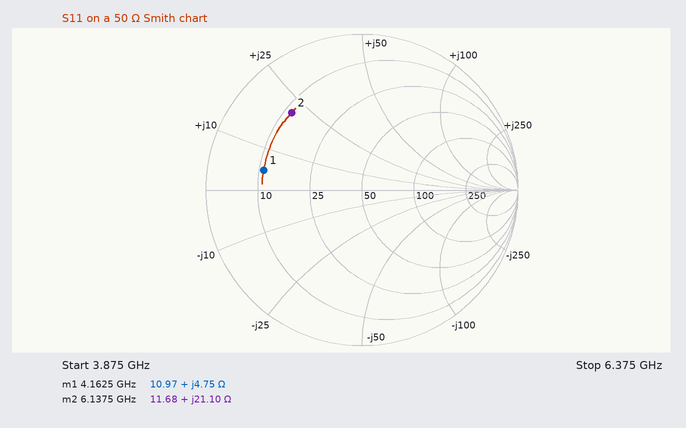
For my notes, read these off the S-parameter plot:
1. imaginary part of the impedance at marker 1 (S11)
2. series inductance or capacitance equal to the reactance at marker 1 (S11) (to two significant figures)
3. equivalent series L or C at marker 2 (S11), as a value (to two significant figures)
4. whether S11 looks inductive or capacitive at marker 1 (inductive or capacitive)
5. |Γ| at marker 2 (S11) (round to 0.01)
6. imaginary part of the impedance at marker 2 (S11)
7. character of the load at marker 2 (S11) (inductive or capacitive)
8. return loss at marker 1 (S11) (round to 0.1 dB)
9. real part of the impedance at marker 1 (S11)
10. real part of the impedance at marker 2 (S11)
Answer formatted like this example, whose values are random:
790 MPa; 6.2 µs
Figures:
+4.75 Ω; 180 pH; 550 pH; inductive; 0.67; +21.10 Ω; inductive; 3.8 dB; 10.97 Ω; 11.68 Ω
